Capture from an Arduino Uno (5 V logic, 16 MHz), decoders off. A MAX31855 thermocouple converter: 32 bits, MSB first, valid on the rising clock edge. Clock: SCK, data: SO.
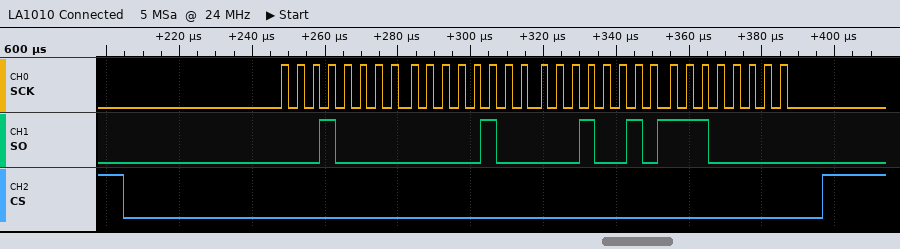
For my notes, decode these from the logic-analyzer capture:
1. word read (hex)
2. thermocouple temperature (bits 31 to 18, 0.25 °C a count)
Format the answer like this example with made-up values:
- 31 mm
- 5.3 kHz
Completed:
- 0x100412E0
- 256.25 °C
